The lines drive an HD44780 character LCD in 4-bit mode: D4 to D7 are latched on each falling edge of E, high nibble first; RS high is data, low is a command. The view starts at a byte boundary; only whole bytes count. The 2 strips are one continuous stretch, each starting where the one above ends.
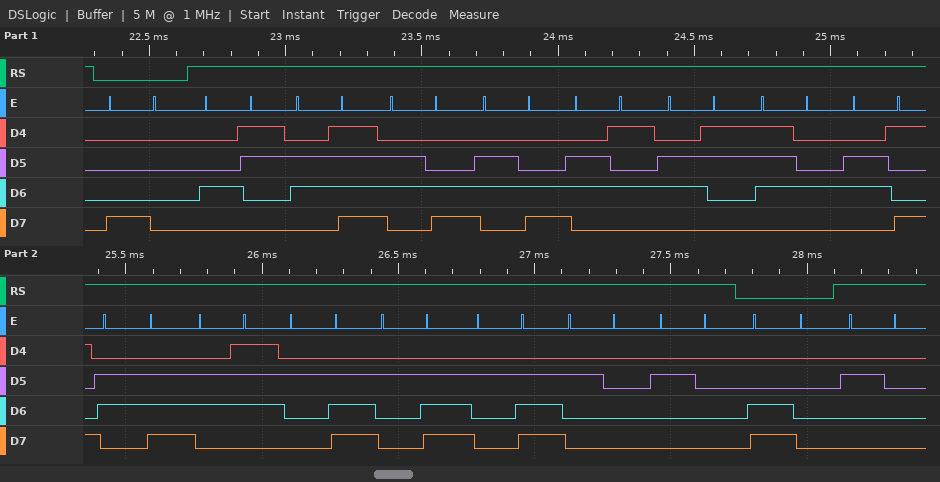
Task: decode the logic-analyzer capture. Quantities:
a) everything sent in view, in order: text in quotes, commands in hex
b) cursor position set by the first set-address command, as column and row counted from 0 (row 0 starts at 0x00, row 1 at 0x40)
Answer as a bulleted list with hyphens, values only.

- 0x80 "Collecting...  " 0xC0 " "
- column 0, row 0
